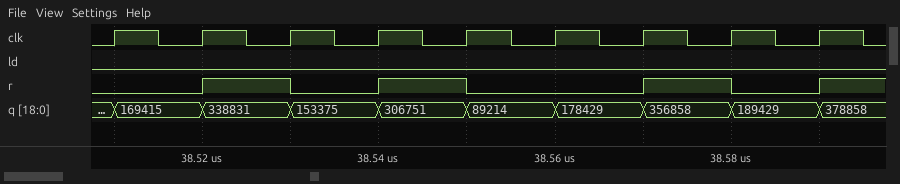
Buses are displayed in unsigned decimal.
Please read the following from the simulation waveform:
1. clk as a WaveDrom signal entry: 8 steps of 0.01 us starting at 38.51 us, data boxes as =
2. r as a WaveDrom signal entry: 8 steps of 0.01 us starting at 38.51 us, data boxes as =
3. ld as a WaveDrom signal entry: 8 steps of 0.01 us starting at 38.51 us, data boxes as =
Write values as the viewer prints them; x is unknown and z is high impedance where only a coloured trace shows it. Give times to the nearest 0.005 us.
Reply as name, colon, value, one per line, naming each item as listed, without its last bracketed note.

clk as a WaveDrom signal entry: 8 steps of 0.01 us starting at 38.51 us, data boxes as =: {name: 'clk', wave: 'p.......'}
r as a WaveDrom signal entry: 8 steps of 0.01 us starting at 38.51 us, data boxes as =: {name: 'r', wave: '01010.10'}
ld as a WaveDrom signal entry: 8 steps of 0.01 us starting at 38.51 us, data boxes as =: {name: 'ld', wave: '0.......'}
